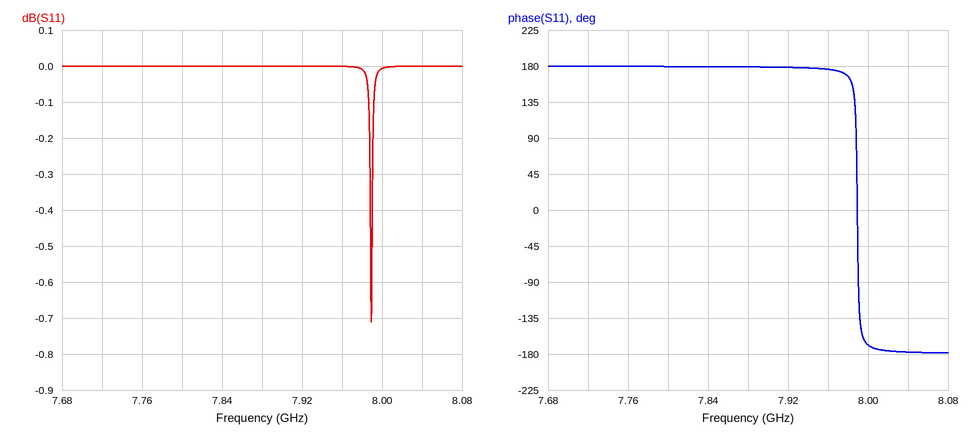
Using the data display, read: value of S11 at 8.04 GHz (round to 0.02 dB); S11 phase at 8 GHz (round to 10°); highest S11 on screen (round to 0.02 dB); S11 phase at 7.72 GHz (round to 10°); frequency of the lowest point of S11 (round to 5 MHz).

0.00 dB
-170°
0.00 dB
180°
7.990 GHz
